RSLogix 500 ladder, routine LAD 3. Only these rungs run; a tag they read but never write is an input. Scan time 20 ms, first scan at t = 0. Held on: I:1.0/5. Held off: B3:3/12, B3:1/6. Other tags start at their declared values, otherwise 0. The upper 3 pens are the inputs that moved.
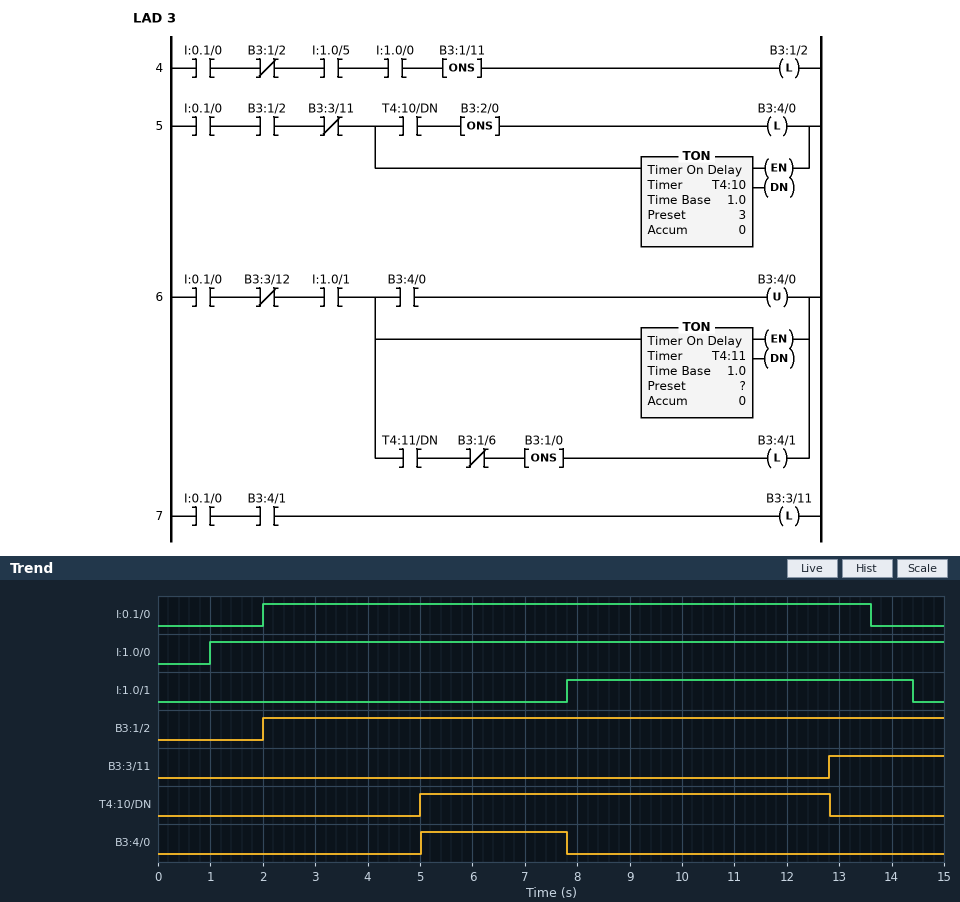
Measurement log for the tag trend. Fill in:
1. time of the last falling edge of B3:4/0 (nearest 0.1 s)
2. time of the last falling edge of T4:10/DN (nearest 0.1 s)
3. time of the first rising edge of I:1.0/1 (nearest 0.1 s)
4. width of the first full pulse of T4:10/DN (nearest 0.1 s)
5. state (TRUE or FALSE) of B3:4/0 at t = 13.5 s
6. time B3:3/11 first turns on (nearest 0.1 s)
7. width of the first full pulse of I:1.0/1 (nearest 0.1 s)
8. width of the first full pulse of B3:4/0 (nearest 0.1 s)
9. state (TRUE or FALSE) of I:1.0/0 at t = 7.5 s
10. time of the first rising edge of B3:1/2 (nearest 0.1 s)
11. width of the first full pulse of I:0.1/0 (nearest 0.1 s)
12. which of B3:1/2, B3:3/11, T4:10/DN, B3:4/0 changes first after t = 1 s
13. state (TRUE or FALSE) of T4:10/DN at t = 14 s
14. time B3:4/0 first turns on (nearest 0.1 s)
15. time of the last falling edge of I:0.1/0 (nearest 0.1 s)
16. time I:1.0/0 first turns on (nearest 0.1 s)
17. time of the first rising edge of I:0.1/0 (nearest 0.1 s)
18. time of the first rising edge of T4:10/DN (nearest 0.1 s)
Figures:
7.8 s
12.8 s
7.8 s
7.8 s
FALSE
12.8 s
6.6 s
2.8 s
TRUE
2.0 s
11.6 s
B3:1/2
FALSE
5.0 s
13.6 s
1.0 s
2.0 s
5.0 s
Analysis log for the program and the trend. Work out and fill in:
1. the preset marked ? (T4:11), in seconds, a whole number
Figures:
5 s
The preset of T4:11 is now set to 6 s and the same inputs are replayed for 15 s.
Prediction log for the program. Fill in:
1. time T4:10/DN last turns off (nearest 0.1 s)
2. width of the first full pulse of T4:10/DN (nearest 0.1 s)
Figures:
13.6 s
8.6 s
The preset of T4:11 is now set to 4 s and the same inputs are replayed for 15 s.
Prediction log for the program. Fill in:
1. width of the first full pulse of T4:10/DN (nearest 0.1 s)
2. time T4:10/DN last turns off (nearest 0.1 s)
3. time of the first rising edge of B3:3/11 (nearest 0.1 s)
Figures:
6.8 s
11.8 s
11.8 s
